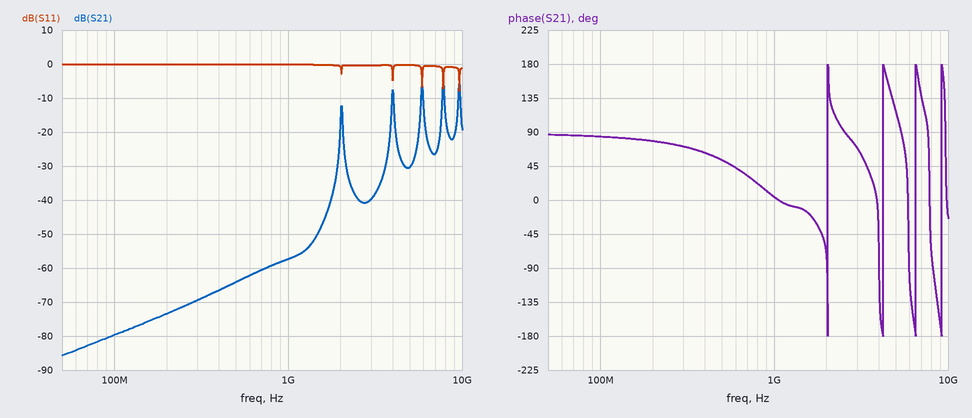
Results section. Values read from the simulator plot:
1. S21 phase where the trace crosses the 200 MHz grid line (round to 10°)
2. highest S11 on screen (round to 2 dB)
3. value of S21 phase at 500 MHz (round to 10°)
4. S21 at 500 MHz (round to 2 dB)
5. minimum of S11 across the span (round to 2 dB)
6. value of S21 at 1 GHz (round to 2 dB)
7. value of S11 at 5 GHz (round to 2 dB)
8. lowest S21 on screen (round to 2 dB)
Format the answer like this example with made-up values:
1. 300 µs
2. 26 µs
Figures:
1. 80°
2. 0 dB
3. 50°
4. -64 dB
5. -8 dB
6. -58 dB
7. 0 dB
8. -86 dB
